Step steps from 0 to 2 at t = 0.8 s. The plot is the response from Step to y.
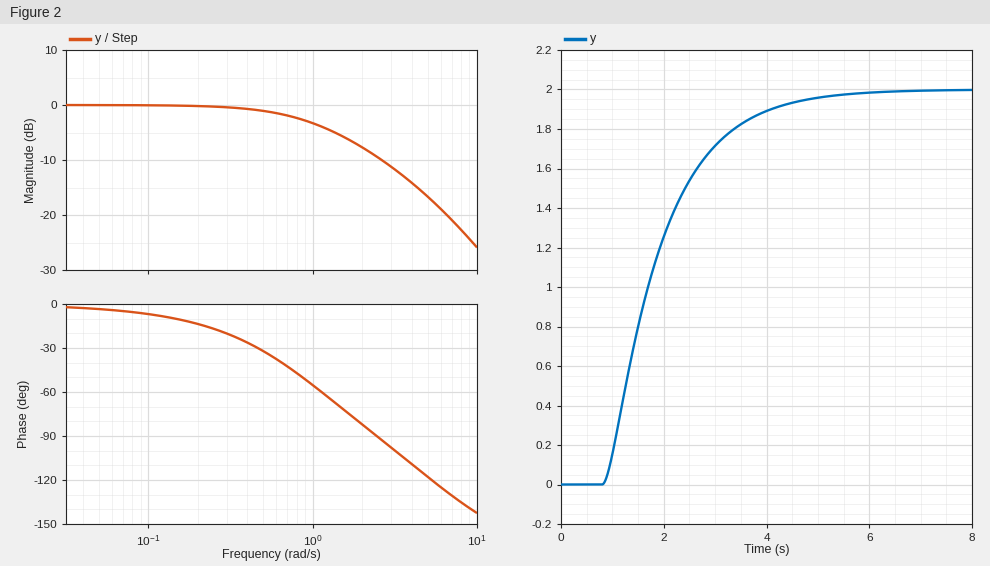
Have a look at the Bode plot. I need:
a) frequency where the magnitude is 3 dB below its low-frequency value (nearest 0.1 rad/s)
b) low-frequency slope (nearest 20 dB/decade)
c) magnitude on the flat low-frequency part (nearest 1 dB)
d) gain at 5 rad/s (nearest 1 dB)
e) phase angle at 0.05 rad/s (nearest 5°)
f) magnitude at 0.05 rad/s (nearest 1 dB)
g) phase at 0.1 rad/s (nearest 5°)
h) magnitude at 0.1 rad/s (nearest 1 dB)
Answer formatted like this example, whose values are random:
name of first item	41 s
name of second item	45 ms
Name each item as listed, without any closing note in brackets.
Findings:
frequency where the magnitude is 3 dB below its low-frequency value	0.9 rad/s
low-frequency slope	0 dB/decade
magnitude on the flat low-frequency part	0 dB
gain at 5 rad/s	-17 dB
phase angle at 0.05 rad/s	-5°
magnitude at 0.05 rad/s	0 dB
phase at 0.1 rad/s	-5°
magnitude at 0.1 rad/s	0 dB
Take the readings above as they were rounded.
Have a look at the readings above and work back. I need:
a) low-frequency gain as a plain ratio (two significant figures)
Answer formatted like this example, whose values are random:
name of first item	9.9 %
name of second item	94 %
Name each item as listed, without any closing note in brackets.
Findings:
low-frequency gain as a plain ratio	1.0
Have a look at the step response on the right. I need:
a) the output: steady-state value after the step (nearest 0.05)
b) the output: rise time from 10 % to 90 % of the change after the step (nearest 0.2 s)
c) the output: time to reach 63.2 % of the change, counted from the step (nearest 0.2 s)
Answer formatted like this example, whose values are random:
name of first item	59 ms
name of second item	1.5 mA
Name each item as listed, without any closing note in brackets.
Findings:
the output: steady-state value after the step	2.00
the output: rise time from 10 % to 90 % of the change after the step	2.4 s
the output: time to reach 63.2 % of the change, counted from the step	1.2 s
